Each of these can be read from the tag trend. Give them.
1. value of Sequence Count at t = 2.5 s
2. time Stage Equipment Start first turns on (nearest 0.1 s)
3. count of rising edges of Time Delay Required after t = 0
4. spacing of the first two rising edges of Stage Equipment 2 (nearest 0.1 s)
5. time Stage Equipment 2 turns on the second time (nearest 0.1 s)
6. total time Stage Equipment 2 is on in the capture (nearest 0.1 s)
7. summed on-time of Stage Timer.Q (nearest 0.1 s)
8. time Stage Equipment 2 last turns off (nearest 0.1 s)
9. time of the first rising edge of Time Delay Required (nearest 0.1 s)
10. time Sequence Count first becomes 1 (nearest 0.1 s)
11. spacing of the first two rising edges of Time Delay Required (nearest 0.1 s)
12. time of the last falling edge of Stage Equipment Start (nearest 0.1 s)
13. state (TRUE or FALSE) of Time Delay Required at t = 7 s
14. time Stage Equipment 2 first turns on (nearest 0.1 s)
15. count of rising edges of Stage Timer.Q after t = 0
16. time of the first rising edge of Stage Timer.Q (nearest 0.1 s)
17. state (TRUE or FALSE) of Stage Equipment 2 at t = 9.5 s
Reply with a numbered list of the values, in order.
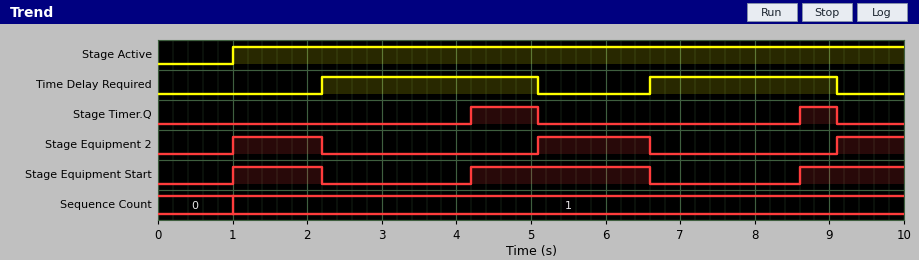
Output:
1. 1
2. 1.0 s
3. 2
4. 4.1 s
5. 5.1 s
6. 3.6 s
7. 1.4 s
8. 6.6 s
9. 2.2 s
10. 1.0 s
11. 4.4 s
12. 6.6 s
13. TRUE
14. 1.0 s
15. 2
16. 4.2 s
17. TRUE
